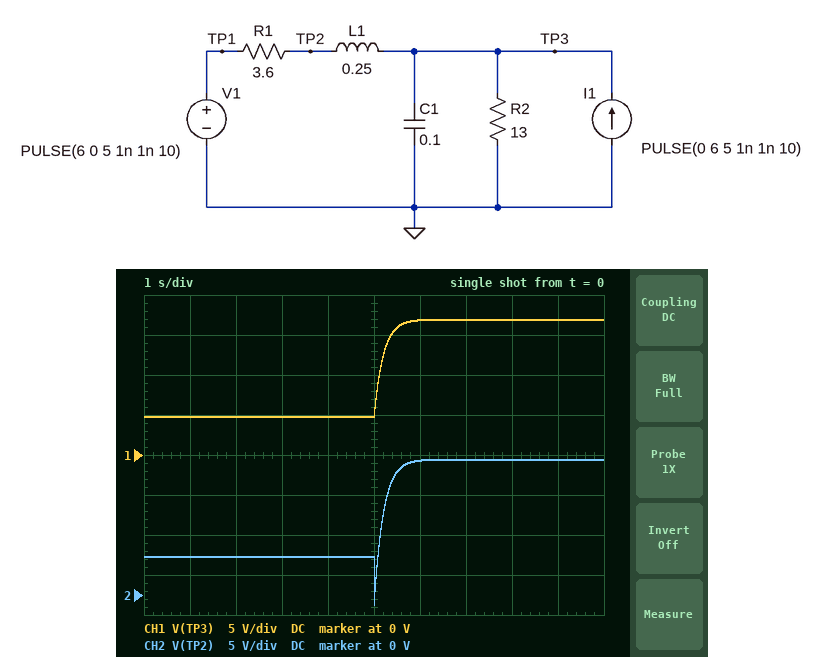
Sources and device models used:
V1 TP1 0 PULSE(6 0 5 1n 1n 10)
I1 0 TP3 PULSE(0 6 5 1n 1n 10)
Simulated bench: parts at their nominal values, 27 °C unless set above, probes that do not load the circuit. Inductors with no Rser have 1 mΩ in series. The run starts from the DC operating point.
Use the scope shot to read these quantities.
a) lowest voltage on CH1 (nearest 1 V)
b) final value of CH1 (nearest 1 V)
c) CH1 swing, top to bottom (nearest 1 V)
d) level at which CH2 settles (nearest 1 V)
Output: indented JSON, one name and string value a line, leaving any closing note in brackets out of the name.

{
  "lowest voltage on CH1": "5 V",
  "final value of CH1": "17 V",
  "CH1 swing, top to bottom": "12 V",
  "level at which CH2 settles": "17 V"
}
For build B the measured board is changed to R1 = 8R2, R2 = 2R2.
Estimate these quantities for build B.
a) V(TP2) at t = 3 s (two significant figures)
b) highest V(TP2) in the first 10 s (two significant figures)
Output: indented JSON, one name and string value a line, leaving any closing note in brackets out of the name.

{
  "V(TP2) at t = 3 s": "1.3 V",
  "highest V(TP2) in the first 10 s": "10 V"
}
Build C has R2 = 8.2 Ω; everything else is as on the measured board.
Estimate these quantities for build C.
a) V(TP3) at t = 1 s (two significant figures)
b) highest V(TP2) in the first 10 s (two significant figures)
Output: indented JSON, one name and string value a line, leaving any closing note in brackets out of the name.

{
  "V(TP3) at t = 1 s": "4.2 V",
  "highest V(TP2) in the first 10 s": "15 V"
}
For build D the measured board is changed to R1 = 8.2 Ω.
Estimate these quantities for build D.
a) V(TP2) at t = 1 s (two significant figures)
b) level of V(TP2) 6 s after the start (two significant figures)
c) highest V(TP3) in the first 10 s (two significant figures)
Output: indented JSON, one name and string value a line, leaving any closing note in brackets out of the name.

{
  "V(TP2) at t = 1 s": "3.7 V",
  "level of V(TP2) 6 s after the start": "27 V",
  "highest V(TP3) in the first 10 s": "30 V"
}
